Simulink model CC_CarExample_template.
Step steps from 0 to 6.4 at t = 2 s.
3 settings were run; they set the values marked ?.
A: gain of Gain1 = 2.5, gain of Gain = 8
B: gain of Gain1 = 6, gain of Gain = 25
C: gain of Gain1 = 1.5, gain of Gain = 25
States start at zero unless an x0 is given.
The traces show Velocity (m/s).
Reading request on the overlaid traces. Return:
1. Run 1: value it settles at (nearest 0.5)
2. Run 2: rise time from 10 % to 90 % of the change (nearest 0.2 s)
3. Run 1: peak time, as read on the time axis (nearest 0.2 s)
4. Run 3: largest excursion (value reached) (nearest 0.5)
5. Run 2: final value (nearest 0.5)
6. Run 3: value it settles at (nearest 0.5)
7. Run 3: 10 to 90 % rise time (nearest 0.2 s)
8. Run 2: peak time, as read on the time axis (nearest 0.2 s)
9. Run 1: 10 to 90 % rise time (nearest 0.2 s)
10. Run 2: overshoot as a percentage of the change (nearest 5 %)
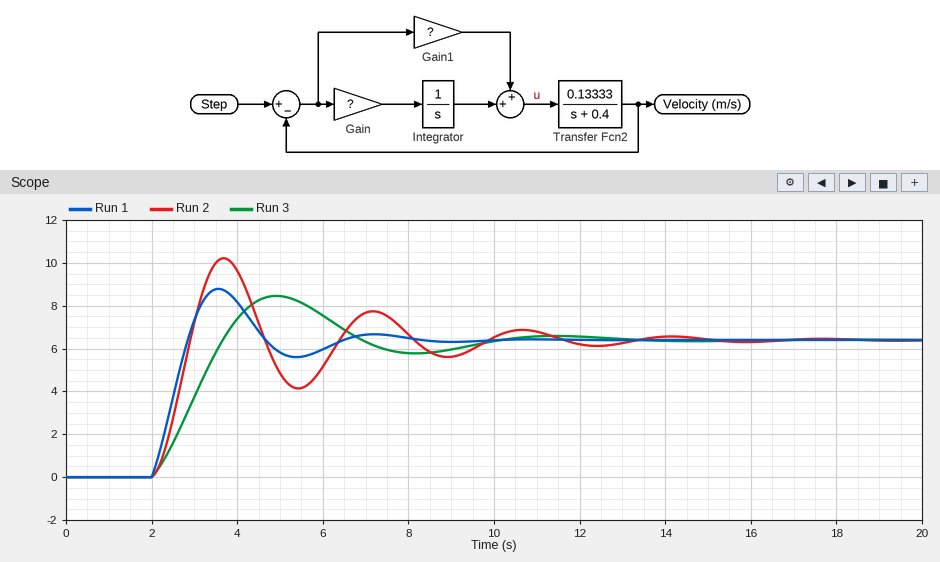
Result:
6.5
0.6 s
3.6 s
8.5
6.5
6.5
1.2 s
3.6 s
0.6 s
60 %
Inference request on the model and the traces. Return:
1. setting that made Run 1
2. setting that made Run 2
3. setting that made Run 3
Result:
B
C
A
